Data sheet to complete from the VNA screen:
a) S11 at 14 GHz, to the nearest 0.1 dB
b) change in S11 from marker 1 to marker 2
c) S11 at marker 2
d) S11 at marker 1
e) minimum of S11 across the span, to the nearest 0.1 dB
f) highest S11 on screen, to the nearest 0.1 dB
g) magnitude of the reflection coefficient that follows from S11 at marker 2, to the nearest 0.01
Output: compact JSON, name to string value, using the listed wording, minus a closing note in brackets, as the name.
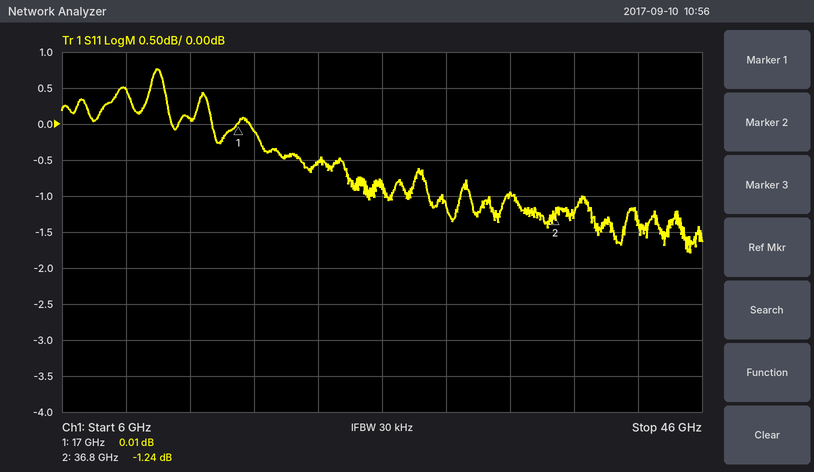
{"S11 at 14 GHz, to the nearest 0.1 dB": "0.1 dB", "change in S11 from marker 1 to marker 2": "-1.25 dB", "S11 at marker 2": "-1.24 dB", "S11 at marker 1": "0.01 dB", "minimum of S11 across the span, to the nearest 0.1 dB": "-1.8 dB", "highest S11 on screen, to the nearest 0.1 dB": "0.8 dB", "magnitude of the reflection coefficient that follows from S11 at marker 2, to the nearest 0.01": "0.87"}
